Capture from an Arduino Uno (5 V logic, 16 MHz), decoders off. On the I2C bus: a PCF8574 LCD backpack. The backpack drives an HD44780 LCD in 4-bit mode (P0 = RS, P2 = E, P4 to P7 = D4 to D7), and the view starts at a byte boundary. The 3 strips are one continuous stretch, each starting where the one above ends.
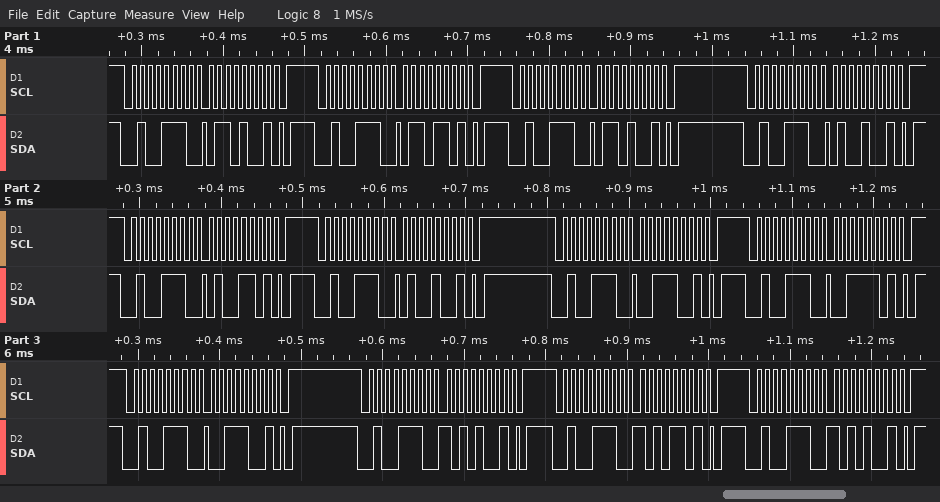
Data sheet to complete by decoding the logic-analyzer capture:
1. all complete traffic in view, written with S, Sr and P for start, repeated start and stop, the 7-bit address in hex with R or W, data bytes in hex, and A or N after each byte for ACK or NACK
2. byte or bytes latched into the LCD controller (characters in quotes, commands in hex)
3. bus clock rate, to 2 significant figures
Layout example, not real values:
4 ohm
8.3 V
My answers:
S 27W A 69 A P S 27W A 6D A P S 27W A 69 A P S 27W A 49 A P S 27W A 4D A P S 27W A 49 A P S 27W A 39 A P S 27W A 3D A P S 27W A 39 A P S 27W A A9 A P S 27W A AD A P S 27W A A9 A P
'd' ':'
100 kHz
